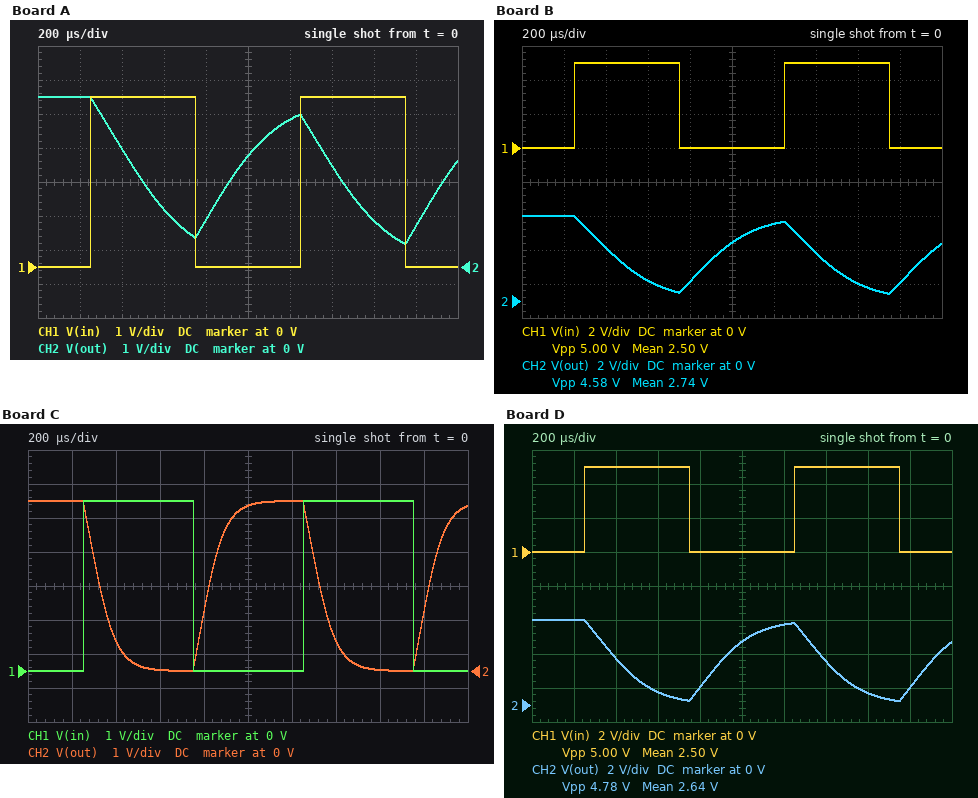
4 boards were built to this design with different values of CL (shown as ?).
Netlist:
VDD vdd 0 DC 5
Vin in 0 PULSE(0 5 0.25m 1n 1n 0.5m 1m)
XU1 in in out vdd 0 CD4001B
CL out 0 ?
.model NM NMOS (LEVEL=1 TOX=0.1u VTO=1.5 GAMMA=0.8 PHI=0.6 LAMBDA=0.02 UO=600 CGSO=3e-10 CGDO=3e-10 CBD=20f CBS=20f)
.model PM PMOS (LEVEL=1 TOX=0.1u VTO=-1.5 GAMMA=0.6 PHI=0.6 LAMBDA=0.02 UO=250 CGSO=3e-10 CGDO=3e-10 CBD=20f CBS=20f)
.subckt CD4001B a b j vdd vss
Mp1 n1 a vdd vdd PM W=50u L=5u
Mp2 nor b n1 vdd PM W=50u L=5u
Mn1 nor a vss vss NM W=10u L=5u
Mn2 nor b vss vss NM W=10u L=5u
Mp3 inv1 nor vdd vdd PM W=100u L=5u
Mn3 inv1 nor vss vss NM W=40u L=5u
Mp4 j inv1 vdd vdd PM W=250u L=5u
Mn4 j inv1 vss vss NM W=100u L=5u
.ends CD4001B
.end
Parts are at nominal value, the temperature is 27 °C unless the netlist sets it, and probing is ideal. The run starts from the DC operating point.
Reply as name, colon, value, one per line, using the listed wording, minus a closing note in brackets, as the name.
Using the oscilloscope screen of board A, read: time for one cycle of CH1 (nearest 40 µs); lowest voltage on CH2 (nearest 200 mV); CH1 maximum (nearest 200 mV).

time for one cycle of CH1: 1.00 ms
lowest voltage on CH2: 600 mV
CH1 maximum: 5.0 V
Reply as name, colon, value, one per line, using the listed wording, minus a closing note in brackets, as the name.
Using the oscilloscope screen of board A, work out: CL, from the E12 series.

CL, from the E12 series: 270 nF
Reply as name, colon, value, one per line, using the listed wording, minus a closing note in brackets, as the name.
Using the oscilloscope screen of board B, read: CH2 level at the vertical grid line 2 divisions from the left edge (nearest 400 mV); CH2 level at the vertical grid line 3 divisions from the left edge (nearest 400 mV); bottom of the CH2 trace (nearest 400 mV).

CH2 level at the vertical grid line 2 divisions from the left edge: 3.2 V
CH2 level at the vertical grid line 3 divisions from the left edge: 1.2 V
bottom of the CH2 trace: 400 mV
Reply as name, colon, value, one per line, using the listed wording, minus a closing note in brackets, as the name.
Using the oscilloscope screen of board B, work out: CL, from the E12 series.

CL, from the E12 series: 220 nF
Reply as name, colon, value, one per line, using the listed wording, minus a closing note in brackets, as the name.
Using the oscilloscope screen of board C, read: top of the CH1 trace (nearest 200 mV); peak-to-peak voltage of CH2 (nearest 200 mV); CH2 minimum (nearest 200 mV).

top of the CH1 trace: 5.0 V
peak-to-peak voltage of CH2: 5.0 V
CH2 minimum: 0 V
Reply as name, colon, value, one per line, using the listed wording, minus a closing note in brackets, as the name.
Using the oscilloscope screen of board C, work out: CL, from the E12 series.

CL, from the E12 series: 82 nF
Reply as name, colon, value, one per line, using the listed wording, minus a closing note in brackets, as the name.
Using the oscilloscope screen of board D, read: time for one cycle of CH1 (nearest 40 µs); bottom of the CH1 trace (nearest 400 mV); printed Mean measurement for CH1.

time for one cycle of CH1: 1.00 ms
bottom of the CH1 trace: 0 V
printed Mean measurement for CH1: 2.50 V
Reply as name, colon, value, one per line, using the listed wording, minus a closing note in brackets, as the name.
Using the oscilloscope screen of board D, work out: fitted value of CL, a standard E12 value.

fitted value of CL, a standard E12 value: 180 nF
